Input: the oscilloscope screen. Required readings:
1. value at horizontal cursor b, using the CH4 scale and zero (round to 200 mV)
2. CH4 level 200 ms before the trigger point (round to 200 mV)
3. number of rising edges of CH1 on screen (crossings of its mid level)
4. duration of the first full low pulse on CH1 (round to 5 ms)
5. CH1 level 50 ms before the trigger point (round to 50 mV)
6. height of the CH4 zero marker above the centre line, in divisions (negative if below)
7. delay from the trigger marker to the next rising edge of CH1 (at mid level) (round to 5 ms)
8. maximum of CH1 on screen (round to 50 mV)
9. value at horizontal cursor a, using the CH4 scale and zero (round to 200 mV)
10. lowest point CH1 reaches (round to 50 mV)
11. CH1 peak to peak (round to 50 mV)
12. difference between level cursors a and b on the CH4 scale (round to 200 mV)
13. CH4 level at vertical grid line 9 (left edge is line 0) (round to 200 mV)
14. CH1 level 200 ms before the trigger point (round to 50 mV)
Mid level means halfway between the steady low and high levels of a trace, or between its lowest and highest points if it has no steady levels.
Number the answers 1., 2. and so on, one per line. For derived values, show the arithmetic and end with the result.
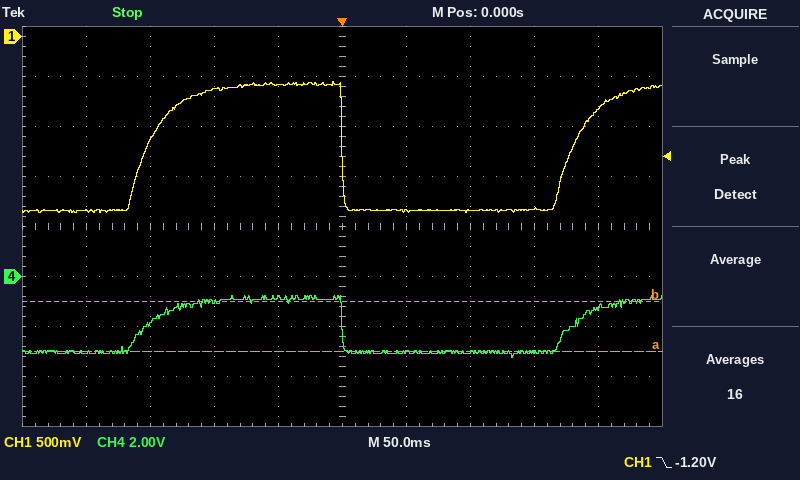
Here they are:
1. -1.0 V
2. -3.0 V
3. 2
4. 180 ms
5. -500 mV
6. -1.0 div
7. 180 ms
8. -450 mV
9. -3.0 V
10. -1.75 V
11. -450 mV − (-1.75 V) = 1.30 V
12. 2.0 V
13. -1.2 V
14. -1.75 V
